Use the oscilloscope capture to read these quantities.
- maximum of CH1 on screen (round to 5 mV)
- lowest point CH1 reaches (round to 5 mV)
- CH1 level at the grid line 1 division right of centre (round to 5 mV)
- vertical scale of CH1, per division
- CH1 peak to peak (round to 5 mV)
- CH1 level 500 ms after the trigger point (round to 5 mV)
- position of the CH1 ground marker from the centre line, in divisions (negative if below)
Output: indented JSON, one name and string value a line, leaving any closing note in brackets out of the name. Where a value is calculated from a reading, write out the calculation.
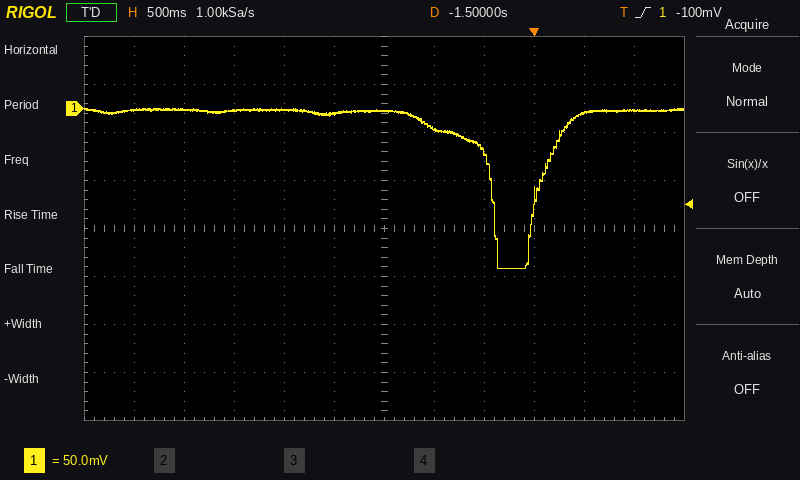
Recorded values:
{
  "maximum of CH1 on screen": "0 mV",
  "lowest point CH1 reaches": "-165 mV",
  "CH1 level at the grid line 1 division right of centre": "-20 mV",
  "vertical scale of CH1, per division": "50 mV",
  "CH1 peak to peak": "0 mV − (-165 mV) = 165 mV",
  "CH1 level 500 ms after the trigger point": "-5 mV",
  "position of the CH1 ground marker from the centre line, in divisions": "+2.5 div"
}
